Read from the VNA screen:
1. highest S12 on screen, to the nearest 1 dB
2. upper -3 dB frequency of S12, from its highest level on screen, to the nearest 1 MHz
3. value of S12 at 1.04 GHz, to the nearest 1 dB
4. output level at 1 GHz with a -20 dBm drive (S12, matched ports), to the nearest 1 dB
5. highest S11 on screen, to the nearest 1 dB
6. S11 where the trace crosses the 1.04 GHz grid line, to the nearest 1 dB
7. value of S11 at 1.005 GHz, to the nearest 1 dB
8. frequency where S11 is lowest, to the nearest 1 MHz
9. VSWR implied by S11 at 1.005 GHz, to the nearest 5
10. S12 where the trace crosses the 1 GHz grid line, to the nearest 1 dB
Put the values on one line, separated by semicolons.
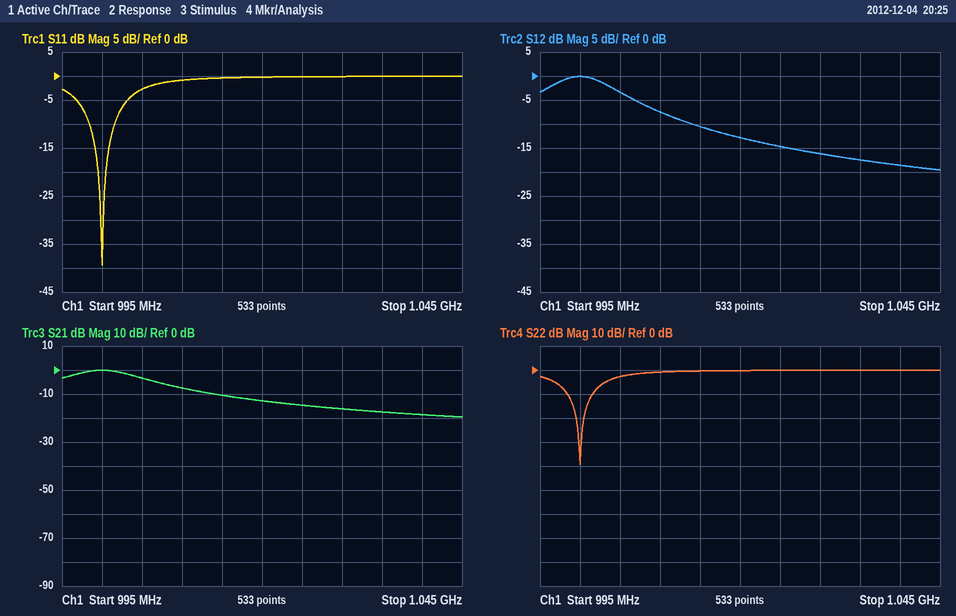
0 dB; 1.005 GHz; -19 dB; -20 dBm; 0 dB; 0 dB; -3 dB; 1.000 GHz; 5; 0 dB
